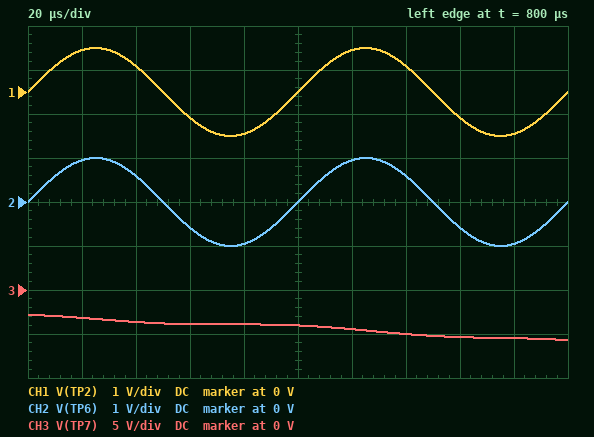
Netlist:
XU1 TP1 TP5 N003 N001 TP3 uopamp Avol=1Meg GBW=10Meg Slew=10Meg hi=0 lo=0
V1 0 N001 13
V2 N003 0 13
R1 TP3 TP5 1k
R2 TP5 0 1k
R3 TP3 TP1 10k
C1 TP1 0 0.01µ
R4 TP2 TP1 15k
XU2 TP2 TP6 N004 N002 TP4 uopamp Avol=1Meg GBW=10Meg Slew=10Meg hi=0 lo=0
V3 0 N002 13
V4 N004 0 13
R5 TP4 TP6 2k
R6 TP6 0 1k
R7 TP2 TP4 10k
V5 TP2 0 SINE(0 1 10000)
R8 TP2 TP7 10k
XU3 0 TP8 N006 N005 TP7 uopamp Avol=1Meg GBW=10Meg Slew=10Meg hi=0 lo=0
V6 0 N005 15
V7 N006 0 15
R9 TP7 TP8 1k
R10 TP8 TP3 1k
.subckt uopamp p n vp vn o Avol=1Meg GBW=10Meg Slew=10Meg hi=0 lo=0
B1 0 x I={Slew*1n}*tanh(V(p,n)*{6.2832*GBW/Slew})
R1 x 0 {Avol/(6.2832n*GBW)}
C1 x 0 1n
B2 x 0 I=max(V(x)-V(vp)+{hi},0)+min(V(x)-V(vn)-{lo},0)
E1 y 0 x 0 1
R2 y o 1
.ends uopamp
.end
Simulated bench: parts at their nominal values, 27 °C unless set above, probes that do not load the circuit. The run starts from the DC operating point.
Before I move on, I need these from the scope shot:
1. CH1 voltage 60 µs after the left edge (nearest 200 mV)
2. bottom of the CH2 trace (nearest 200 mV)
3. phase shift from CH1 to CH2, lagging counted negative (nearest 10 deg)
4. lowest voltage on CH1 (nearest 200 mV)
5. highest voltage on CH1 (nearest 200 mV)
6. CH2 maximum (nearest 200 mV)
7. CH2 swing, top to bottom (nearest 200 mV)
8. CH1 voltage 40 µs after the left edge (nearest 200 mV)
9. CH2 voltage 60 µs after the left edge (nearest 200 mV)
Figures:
-600 mV
-1.0 V
0 deg
-1.0 V
1.0 V
1.0 V
2.0 V
600 mV
-600 mV
